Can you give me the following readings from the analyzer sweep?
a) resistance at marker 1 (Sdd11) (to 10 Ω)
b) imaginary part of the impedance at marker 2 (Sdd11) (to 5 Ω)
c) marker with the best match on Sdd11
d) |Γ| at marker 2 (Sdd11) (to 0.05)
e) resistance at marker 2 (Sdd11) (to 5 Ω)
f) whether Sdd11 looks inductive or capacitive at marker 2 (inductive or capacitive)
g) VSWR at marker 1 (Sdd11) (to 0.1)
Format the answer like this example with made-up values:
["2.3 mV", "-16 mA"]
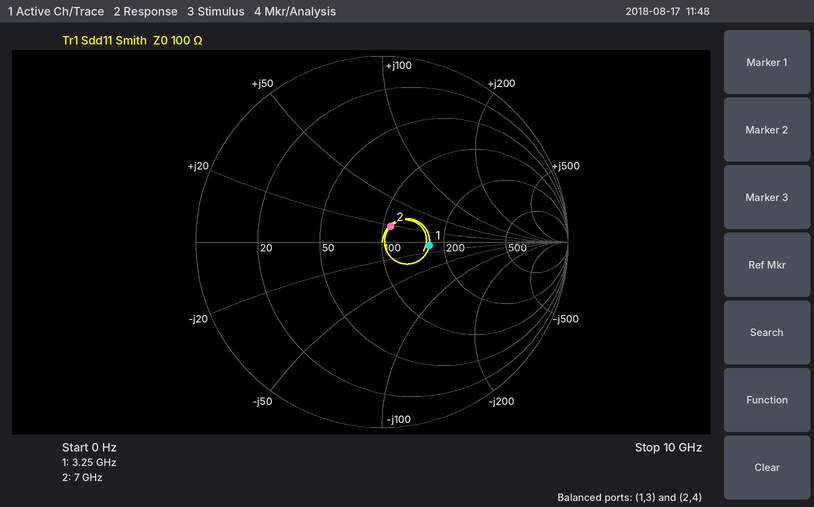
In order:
["170 Ω", "+20 Ω", "marker 2", "0.10", "110 Ω", "inductive", "1.7"]
